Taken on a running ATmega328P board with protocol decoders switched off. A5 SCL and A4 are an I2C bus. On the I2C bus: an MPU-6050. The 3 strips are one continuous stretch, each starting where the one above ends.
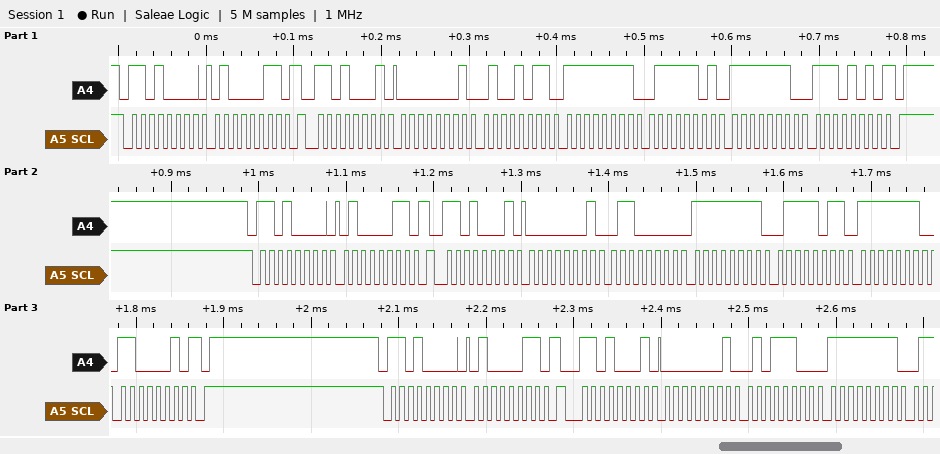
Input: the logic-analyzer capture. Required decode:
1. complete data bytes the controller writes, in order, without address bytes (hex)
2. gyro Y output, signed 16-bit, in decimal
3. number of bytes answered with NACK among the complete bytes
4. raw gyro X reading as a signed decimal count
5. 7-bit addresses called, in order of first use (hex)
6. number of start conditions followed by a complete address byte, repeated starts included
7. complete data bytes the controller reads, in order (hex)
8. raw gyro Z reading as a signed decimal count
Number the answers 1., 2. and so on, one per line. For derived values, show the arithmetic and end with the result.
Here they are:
1. 43 43 43
2. 0xFF7D = -131
3. 2
4. 0x014B = 331
5. 0x68
6. 6
7. 01 4B FF 7D FE EA 01 60 FF 7B FE C2 01 5C FF
8. 0xFEEA = -278
